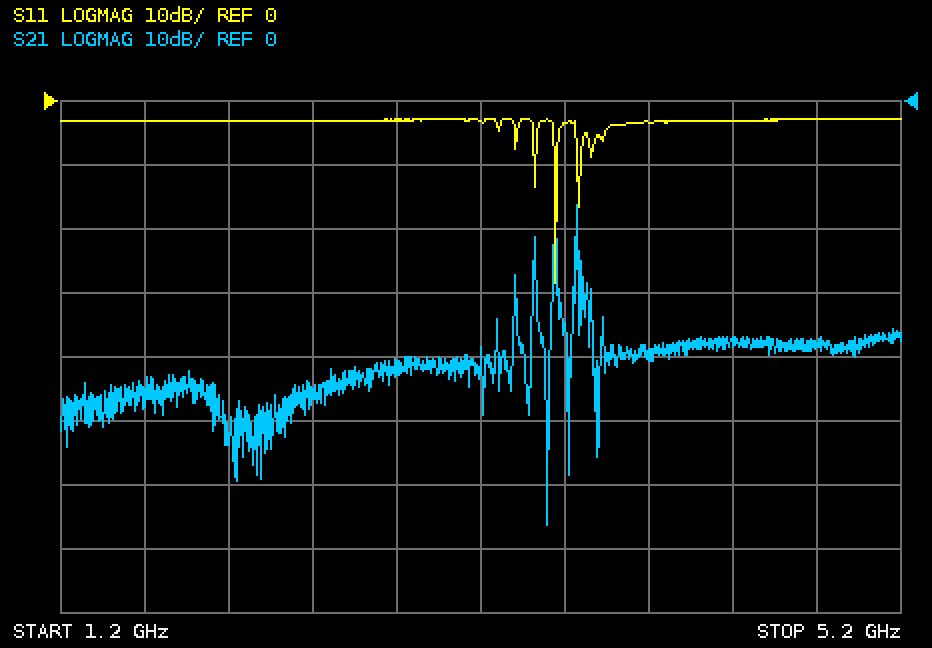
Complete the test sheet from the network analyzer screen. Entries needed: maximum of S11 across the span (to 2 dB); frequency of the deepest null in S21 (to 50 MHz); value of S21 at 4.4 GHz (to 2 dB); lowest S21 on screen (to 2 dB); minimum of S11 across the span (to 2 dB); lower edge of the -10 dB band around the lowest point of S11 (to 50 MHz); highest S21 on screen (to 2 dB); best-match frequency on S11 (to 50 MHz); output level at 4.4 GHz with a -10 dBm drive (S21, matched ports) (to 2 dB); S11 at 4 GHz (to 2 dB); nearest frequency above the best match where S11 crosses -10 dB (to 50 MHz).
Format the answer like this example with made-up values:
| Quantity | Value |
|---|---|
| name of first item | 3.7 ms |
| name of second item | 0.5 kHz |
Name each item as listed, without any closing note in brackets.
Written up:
| Quantity | Value |
|---|---|
| maximum of S11 across the span | -2 dB |
| frequency of the deepest null in S21 | 3.50 GHz |
| value of S21 at 4.4 GHz | -38 dB |
| lowest S21 on screen | -66 dB |
| minimum of S11 across the span | -28 dB |
| lower edge of the -10 dB band around the lowest point of S11 | 3.55 GHz |
| highest S21 on screen | -16 dB |
| best-match frequency on S11 | 3.55 GHz |
| output level at 4.4 GHz with a -10 dBm drive (S21, matched ports) | -48 dBm |
| S11 at 4 GHz | -4 dB |
| nearest frequency above the best match where S11 crosses -10 dB | 3.55 GHz |
